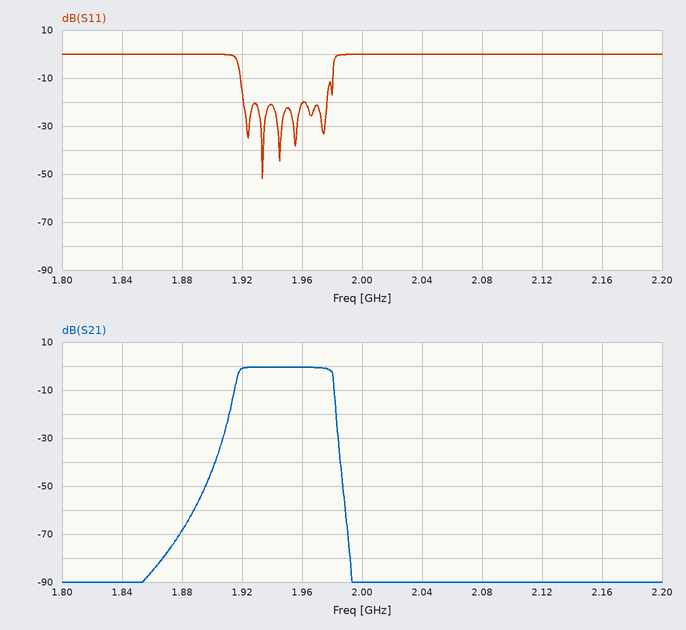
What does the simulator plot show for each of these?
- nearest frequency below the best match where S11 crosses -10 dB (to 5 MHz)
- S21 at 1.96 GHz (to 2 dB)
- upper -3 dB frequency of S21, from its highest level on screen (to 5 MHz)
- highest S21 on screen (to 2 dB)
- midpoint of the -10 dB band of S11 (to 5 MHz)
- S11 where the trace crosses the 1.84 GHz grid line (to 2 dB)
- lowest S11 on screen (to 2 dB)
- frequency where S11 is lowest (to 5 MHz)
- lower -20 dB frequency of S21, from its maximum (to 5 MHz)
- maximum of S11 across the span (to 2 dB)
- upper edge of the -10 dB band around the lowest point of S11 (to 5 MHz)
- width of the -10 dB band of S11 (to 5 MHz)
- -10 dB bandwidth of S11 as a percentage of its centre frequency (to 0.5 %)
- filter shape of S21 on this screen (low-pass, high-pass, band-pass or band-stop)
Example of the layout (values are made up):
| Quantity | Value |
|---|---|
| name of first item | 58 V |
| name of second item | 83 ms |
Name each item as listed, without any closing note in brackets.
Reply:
| Quantity | Value |
|---|---|
| nearest frequency below the best match where S11 crosses -10 dB | 1.920 GHz |
| S21 at 1.96 GHz | 0 dB |
| upper -3 dB frequency of S21, from its highest level on screen | 1.980 GHz |
| highest S21 on screen | 0 dB |
| midpoint of the -10 dB band of S11 | 1.950 GHz |
| S11 where the trace crosses the 1.84 GHz grid line | 0 dB |
| lowest S11 on screen | -52 dB |
| frequency where S11 is lowest | 1.935 GHz |
| lower -20 dB frequency of S21, from its maximum | 1.910 GHz |
| maximum of S11 across the span | 0 dB |
| upper edge of the -10 dB band around the lowest point of S11 | 1.980 GHz |
| width of the -10 dB band of S11 | 60 MHz |
| -10 dB bandwidth of S11 as a percentage of its centre frequency | 3.0 % |
| filter shape of S21 on this screen | band-pass |
